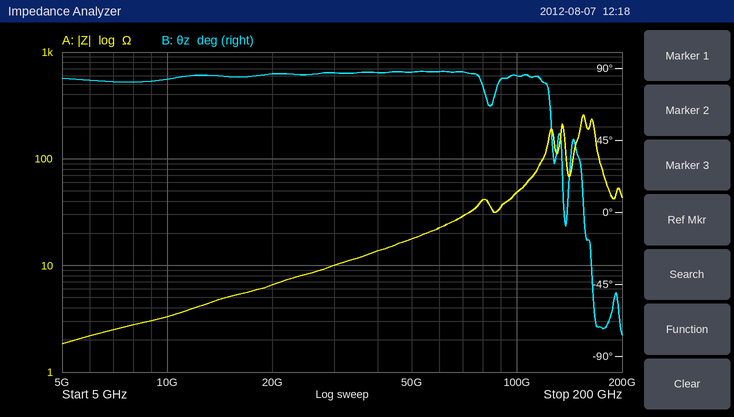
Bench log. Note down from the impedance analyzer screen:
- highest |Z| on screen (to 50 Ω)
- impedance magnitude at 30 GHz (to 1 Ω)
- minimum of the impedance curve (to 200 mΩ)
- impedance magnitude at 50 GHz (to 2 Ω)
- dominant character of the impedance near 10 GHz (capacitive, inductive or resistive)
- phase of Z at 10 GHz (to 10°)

250 Ω
10 Ω
1.8 Ω
18 Ω
inductive
80°
